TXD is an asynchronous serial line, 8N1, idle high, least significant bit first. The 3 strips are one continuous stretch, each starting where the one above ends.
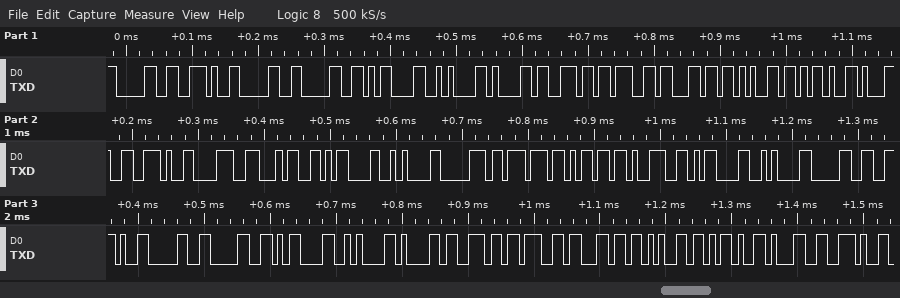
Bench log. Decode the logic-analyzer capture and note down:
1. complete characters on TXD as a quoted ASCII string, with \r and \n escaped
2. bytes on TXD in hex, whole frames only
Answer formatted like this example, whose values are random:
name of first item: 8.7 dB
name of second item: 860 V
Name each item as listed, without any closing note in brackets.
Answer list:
complete characters on TXD as a quoted ASCII string, with \r and \n escaped: "0.00\r\nangle-1.84\r\npwm9\r\n0.00\r\nangle-1."
bytes on TXD in hex, whole frames only: 30 2E 30 30 0D 0A 61 6E 67 6C 65 2D 31 2E 38 34 0D 0A 70 77 6D 39 0D 0A 30 2E 30 30 0D 0A 61 6E 67 6C 65 2D 31 2E
